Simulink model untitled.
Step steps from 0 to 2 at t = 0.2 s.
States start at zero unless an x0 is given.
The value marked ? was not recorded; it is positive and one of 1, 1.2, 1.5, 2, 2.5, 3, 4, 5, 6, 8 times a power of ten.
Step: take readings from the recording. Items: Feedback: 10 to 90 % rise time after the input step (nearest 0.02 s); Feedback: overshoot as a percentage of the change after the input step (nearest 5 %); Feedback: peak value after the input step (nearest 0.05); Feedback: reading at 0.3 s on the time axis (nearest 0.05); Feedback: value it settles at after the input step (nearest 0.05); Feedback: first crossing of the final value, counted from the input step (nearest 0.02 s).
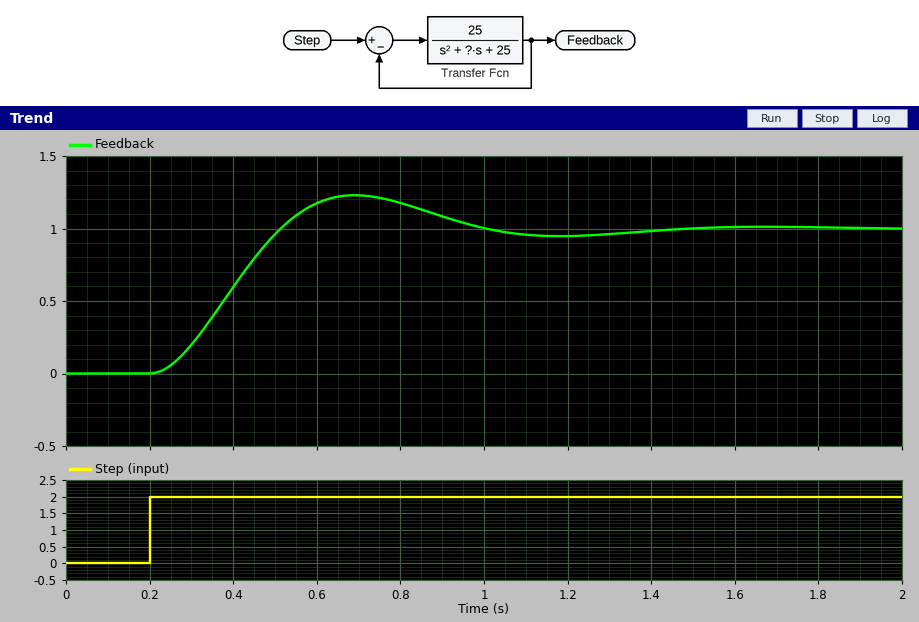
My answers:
0.22 s
25 %
1.25
0.20
1.00
0.32 s
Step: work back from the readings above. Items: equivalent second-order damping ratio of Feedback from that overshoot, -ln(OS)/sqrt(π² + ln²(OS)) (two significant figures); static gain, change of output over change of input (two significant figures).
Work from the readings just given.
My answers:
0.40
0.50
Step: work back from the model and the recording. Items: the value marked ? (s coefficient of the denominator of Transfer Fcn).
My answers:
6
